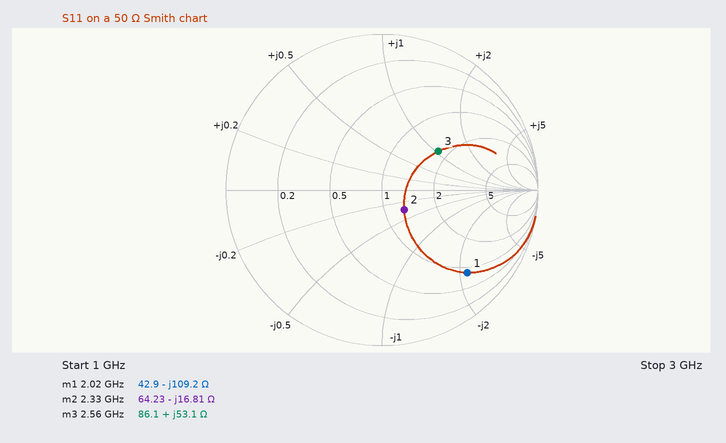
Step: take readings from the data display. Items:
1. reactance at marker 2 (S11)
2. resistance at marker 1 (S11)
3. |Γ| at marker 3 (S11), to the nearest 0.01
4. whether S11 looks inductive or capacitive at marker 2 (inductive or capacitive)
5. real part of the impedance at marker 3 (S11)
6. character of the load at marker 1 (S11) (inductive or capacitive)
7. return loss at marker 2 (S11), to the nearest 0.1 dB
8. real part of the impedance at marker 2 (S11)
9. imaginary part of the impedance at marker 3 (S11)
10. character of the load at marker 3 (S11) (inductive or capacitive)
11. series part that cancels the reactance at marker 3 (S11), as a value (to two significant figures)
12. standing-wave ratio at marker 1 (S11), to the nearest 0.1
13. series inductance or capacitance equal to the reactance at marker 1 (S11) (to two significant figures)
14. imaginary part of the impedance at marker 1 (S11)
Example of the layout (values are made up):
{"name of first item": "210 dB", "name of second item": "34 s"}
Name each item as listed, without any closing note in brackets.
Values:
{"reactance at marker 2": "-16.81 Ω", "resistance at marker 1": "42.9 Ω", "|Γ| at marker 3 (S11), to the nearest 0.01": "0.44", "whether S11 looks inductive or capacitive at marker 2": "capacitive", "real part of the impedance at marker 3": "86.1 Ω", "character of the load at marker 1 (S11)": "capacitive", "return loss at marker 2 (S11), to the nearest 0.1 dB": "14.4 dB", "real part of the impedance at marker 2": "64.23 Ω", "imaginary part of the impedance at marker 3": "+53.1 Ω", "character of the load at marker 3 (S11)": "inductive", "series part that cancels the reactance at marker 3 (S11), as a value": "1.2 pF", "standing-wave ratio at marker 1 (S11), to the nearest 0.1": "7.4", "series inductance or capacitance equal to the reactance at marker 1 (S11)": "720 fF", "imaginary part of the impedance at marker 1": "-109.2 Ω"}
